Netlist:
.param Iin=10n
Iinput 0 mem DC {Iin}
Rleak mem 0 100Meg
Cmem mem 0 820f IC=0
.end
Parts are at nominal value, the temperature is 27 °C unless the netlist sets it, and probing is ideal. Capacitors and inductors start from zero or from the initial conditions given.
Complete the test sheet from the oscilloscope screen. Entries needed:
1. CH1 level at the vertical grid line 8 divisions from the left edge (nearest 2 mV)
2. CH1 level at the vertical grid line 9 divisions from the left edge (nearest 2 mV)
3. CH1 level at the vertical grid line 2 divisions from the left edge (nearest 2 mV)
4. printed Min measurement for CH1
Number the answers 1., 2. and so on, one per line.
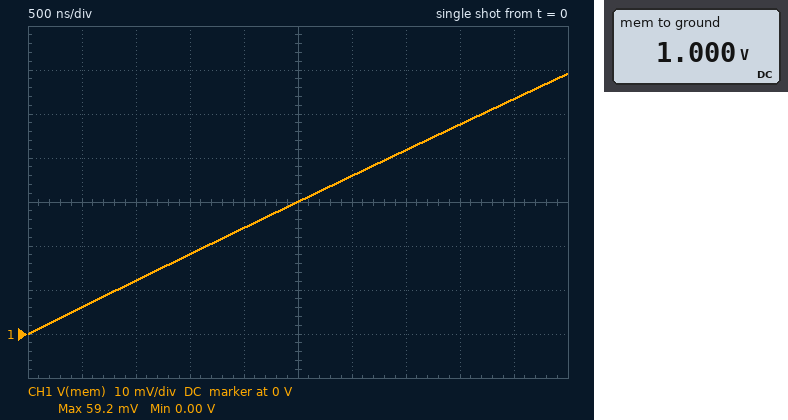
1. 48 mV
2. 54 mV
3. 12 mV
4. 0.00 V
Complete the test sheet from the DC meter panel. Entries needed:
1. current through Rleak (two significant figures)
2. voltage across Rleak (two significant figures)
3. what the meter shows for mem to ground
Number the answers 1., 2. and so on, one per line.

1. 10 nA
2. 1.0 V
3. 1.000 V
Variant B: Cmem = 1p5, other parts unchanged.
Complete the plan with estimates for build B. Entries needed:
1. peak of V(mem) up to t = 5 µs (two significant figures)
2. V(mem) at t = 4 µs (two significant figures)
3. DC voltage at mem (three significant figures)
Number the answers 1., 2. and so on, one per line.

1. 33 mV
2. 26 mV
3. 1.00 V
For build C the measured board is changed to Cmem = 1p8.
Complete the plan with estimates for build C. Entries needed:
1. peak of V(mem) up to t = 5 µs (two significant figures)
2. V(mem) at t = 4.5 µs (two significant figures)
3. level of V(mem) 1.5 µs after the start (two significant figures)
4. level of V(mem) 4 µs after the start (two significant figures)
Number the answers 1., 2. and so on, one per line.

1. 27 mV
2. 25 mV
3. 8.3 mV
4. 22 mV
